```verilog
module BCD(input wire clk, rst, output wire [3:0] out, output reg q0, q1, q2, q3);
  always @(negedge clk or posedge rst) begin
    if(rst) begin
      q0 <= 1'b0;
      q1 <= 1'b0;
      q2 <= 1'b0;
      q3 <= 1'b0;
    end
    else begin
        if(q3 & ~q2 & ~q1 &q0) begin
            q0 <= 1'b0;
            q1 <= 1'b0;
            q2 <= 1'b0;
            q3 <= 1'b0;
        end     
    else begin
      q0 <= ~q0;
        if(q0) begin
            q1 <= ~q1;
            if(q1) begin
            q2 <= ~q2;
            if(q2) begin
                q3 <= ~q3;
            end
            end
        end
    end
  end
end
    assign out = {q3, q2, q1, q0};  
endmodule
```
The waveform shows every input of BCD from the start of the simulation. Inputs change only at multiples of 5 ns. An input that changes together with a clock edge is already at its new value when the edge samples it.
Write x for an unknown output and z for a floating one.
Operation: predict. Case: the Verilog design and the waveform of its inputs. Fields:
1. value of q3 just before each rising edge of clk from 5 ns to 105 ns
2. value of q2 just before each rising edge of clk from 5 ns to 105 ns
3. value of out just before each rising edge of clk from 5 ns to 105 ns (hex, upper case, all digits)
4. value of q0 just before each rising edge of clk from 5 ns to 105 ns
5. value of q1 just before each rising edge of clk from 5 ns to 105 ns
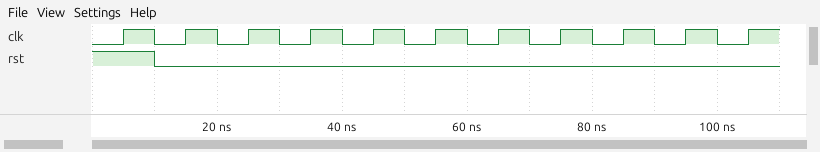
0 0 0 0 0 0 0 0 1 1 0
0 0 0 0 1 1 1 1 0 0 0
0, 1, 2, 3, 4, 5, 6, 7, 8, 9, 0
0 1 0 1 0 1 0 1 0 1 0
0 0 1 1 0 0 1 1 0 0 0
